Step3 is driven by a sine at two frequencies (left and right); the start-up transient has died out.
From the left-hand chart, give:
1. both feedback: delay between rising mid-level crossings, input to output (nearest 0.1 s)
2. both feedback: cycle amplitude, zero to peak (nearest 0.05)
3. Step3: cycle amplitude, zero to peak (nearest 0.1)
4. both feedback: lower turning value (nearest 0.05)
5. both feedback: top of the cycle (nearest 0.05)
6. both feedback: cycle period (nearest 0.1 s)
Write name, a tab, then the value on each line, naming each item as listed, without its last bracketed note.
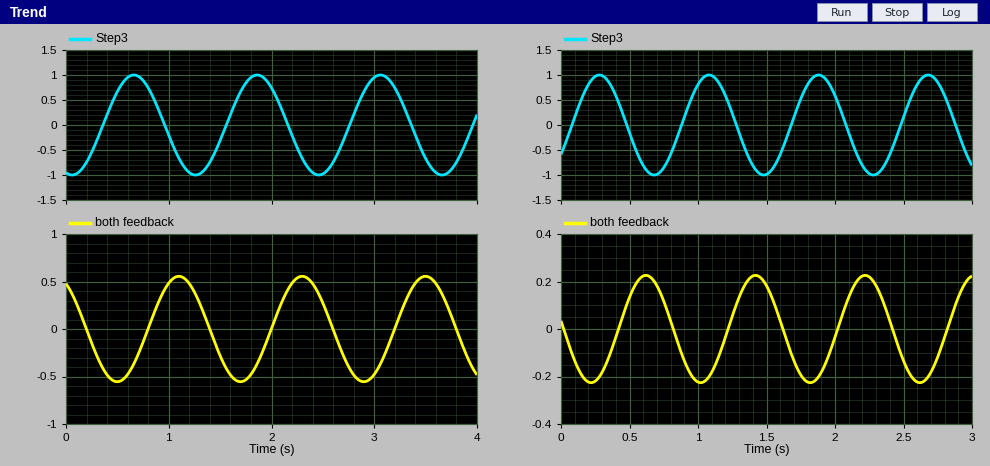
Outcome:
both feedback: delay between rising mid-level crossings, input to output	0.4 s
both feedback: cycle amplitude, zero to peak	0.55
Step3: cycle amplitude, zero to peak	1.0
both feedback: lower turning value	-0.55
both feedback: top of the cycle	0.55
both feedback: cycle period	1.2 s
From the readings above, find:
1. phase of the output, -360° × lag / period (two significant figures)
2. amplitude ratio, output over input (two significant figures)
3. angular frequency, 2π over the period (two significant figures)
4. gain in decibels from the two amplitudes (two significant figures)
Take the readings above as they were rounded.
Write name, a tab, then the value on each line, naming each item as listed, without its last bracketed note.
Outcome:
phase of the output, -360° × lag / period	-120°
amplitude ratio, output over input	0.55
angular frequency, 2π over the period	5.2 rad/s
gain in decibels from the two amplitudes	-5.2 dB
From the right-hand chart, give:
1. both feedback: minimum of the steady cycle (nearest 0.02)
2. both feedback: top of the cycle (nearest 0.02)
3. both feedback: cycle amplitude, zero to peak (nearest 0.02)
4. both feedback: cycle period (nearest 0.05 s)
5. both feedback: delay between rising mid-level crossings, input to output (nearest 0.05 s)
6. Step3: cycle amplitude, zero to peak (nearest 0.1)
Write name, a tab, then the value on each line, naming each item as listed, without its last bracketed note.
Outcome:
both feedback: minimum of the steady cycle	-0.22
both feedback: top of the cycle	0.22
both feedback: cycle amplitude, zero to peak	0.22
both feedback: cycle period	0.80 s
both feedback: delay between rising mid-level crossings, input to output	0.35 s
Step3: cycle amplitude, zero to peak	1.0
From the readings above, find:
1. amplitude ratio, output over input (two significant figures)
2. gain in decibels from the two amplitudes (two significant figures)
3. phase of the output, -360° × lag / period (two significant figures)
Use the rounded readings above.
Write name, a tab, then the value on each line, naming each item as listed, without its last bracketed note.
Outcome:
amplitude ratio, output over input	0.22
gain in decibels from the two amplitudes	-13 dB
phase of the output, -360° × lag / period	-160°
